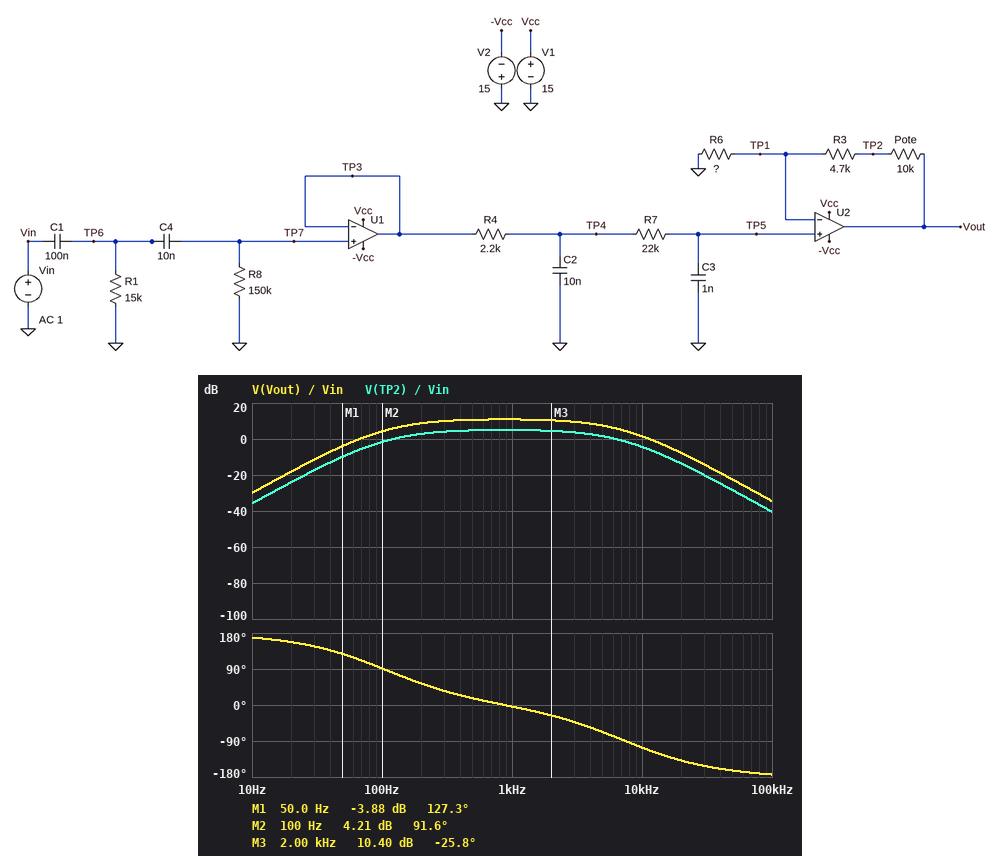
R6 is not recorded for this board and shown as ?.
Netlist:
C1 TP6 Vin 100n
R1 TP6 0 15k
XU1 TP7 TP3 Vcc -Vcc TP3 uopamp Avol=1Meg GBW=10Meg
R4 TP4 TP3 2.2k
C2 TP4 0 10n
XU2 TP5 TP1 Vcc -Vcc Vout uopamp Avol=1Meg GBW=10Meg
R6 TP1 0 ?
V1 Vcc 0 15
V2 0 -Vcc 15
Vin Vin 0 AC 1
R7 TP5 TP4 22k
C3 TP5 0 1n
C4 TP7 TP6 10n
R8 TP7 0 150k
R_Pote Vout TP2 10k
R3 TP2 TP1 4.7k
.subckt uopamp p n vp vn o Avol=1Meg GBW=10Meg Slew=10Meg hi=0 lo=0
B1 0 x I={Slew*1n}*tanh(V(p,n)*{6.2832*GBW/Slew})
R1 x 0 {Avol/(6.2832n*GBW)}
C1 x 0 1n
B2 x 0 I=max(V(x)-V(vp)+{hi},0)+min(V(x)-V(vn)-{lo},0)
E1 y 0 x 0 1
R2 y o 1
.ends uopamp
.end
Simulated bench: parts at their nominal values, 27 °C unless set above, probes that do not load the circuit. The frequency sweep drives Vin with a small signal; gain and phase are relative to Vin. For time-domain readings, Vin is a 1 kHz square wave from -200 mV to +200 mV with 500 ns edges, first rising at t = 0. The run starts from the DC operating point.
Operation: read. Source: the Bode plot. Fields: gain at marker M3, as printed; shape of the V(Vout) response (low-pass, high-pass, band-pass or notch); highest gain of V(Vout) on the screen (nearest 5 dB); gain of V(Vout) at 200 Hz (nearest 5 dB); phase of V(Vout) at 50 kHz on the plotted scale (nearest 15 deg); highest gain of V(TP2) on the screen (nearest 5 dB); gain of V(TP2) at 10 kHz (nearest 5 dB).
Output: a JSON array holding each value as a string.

["10.40 dB", "band-pass", "10 dB", "10 dB", "-165 deg", "5 dB", "-5 dB"]
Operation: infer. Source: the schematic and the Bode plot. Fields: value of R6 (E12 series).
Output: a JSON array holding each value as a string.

["5.6 kΩ"]
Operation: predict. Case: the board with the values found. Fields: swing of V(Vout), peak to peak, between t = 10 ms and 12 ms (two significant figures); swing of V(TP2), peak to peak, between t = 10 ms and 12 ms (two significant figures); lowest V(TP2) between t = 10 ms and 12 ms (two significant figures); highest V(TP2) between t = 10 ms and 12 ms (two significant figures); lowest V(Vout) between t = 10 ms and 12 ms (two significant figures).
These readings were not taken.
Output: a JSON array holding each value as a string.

["1.7 V", "840 mV", "-420 mV", "420 mV", "-830 mV"]
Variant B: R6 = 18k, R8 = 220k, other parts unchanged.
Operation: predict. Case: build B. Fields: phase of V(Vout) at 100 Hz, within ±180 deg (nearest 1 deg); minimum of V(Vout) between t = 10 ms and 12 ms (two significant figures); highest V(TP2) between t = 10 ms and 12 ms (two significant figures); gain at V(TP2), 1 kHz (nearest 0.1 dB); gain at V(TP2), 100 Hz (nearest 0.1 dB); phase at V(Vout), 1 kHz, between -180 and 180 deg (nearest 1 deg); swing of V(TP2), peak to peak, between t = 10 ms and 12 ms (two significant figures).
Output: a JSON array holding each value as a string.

["81 deg", "-410 mV", "280 mV", "1.7 dB", "-3.4 dB", "-6 deg", "560 mV"]
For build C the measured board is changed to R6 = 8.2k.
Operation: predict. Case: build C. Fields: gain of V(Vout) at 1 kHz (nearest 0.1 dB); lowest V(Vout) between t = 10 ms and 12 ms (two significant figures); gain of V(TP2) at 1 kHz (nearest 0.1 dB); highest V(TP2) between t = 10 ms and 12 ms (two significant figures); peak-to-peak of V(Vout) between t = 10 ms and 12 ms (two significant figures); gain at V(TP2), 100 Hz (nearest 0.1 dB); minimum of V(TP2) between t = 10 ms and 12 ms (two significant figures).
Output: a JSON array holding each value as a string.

["8.6 dB", "-640 mV", "3.6 dB", "360 mV", "1.3 V", "-3.0 dB", "-360 mV"]
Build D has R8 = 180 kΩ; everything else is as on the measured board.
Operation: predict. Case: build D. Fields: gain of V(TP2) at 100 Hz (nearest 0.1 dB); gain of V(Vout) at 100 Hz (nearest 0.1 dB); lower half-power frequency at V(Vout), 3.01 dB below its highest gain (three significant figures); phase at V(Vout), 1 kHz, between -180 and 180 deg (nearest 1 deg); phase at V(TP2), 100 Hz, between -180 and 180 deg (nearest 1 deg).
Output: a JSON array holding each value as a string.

["-0.9 dB", "5.0 dB", "153 Hz", "-5 deg", "87 deg"]
